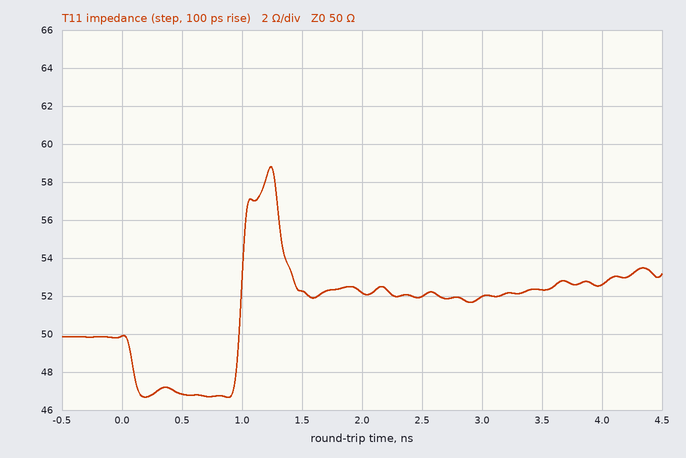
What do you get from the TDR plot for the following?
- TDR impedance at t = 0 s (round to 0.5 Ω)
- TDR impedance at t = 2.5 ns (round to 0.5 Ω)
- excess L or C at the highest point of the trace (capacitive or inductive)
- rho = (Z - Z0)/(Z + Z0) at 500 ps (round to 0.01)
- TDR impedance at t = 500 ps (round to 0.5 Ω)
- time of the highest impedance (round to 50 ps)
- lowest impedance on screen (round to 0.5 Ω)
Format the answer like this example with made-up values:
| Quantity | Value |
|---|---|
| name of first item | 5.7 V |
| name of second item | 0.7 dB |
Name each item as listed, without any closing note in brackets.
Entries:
| Quantity | Value |
|---|---|
| TDR impedance at t = 0 s | 50.0 Ω |
| TDR impedance at t = 2.5 ns | 52.0 Ω |
| excess L or C at the highest point of the trace | inductive |
| rho = (Z - Z0)/(Z + Z0) at 500 ps | -0.03 |
| TDR impedance at t = 500 ps | 47.0 Ω |
| time of the highest impedance | 1.25 ns |
| lowest impedance on screen | 46.5 Ω |
